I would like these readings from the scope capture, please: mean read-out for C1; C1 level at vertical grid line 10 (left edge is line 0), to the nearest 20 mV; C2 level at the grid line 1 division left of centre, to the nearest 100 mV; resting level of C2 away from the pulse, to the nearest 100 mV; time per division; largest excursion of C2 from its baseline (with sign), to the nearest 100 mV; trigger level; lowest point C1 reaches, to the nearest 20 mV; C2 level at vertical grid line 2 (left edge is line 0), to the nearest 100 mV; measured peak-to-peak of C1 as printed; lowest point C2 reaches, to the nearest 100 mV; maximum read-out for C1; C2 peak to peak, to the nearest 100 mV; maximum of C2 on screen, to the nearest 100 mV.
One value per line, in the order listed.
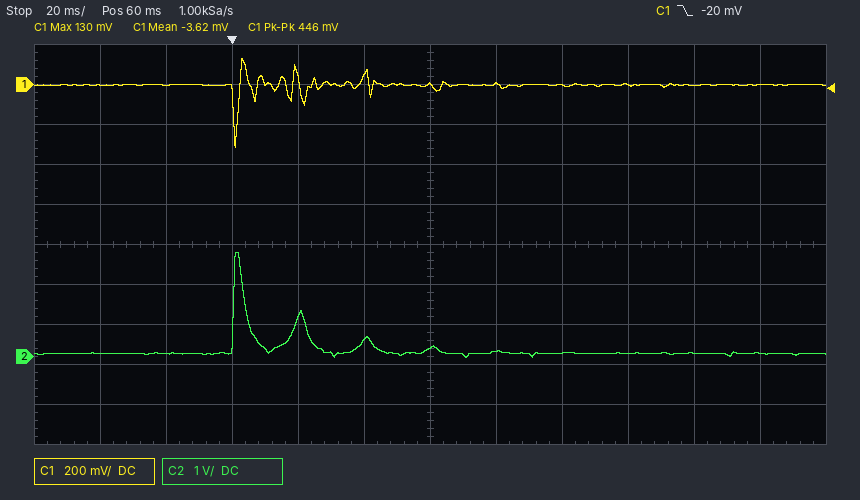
-3.62 mV
0 mV
400 mV
100 mV
20 ms
+2.5 V
-20 mV
-320 mV
100 mV
446 mV
0.0 V
130 mV
2.6 V
2.6 V
